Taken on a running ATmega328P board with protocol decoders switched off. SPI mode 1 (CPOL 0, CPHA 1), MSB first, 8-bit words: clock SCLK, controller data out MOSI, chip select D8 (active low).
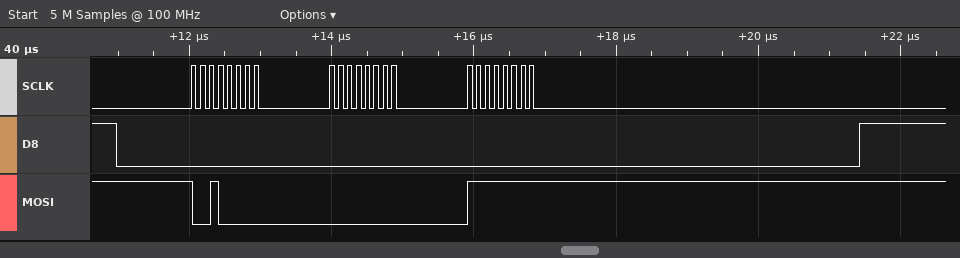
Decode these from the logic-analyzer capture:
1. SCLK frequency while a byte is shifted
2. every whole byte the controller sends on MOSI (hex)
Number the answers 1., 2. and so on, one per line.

1. 8 MHz
2. 0x20 0x00 0xFF
